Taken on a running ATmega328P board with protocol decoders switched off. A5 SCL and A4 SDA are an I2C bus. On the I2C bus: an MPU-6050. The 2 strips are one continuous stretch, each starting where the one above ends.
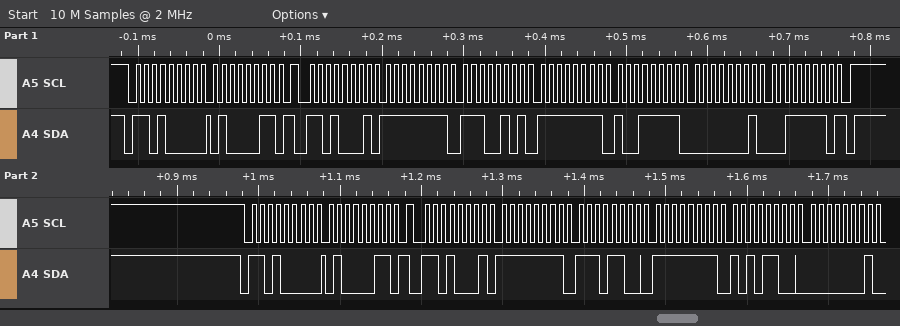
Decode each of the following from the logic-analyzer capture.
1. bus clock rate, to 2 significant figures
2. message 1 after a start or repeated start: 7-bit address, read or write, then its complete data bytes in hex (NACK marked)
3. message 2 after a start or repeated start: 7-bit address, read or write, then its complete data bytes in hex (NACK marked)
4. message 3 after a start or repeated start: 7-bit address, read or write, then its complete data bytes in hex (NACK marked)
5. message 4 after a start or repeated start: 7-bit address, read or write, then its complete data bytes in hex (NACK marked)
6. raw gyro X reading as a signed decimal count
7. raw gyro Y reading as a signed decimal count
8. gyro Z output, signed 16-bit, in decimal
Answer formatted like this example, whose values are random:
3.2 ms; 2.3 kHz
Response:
100 kHz; 0x68 write: 43; 0x68 read: FF E5 FF 9F 01 3E NACK; 0x68 write: 43; 0x68 read: FF EC FF AC 01; -27; -97; 318
